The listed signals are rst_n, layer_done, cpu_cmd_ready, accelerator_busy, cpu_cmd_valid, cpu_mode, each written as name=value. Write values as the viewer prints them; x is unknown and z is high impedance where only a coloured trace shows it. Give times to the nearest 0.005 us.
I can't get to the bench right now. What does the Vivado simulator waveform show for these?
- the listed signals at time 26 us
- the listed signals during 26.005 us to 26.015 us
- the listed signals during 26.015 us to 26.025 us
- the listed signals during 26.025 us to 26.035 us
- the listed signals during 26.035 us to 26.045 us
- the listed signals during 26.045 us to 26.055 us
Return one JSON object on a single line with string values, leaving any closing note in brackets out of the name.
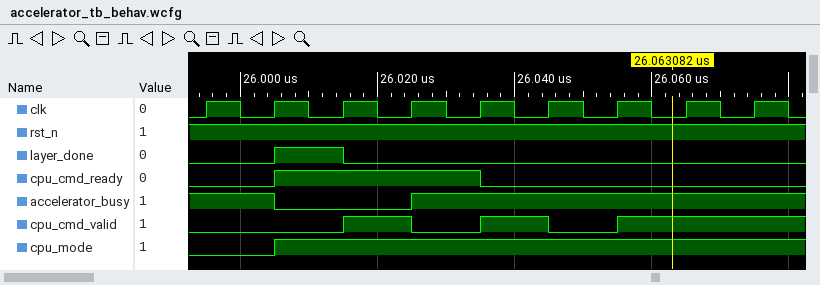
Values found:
{"the listed signals at time 26 us": "rst_n=1, layer_done=0, cpu_cmd_ready=0, accelerator_busy=1, cpu_cmd_valid=0, cpu_mode=0", "the listed signals during 26.005 us to 26.015 us": "rst_n=1, layer_done=1, cpu_cmd_ready=1, accelerator_busy=0, cpu_cmd_valid=0, cpu_mode=1", "the listed signals during 26.015 us to 26.025 us": "rst_n=1, layer_done=0, cpu_cmd_ready=1, accelerator_busy=0, cpu_cmd_valid=1, cpu_mode=1", "the listed signals during 26.025 us to 26.035 us": "rst_n=1, layer_done=0, cpu_cmd_ready=1, accelerator_busy=1, cpu_cmd_valid=0, cpu_mode=1", "the listed signals during 26.035 us to 26.045 us": "rst_n=1, layer_done=0, cpu_cmd_ready=0, accelerator_busy=1, cpu_cmd_valid=1, cpu_mode=1", "the listed signals during 26.045 us to 26.055 us": "rst_n=1, layer_done=0, cpu_cmd_ready=0, accelerator_busy=1, cpu_cmd_valid=0, cpu_mode=1"}
